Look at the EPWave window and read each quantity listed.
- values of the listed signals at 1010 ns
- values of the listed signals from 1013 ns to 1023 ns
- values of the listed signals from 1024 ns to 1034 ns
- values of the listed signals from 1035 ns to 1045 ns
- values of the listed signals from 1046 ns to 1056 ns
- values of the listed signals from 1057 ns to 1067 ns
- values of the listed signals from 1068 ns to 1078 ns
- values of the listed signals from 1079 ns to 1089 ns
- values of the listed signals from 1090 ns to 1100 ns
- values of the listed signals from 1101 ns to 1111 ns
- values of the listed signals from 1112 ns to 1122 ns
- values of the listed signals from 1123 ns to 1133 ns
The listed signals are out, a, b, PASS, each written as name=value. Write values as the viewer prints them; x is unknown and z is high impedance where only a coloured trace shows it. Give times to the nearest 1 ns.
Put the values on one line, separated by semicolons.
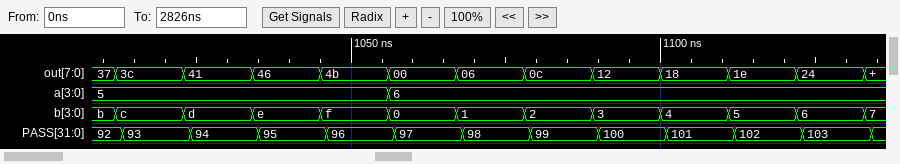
out=37, a=5, b=b, PASS=92; out=3c, a=5, b=c, PASS=93; out=41, a=5, b=d, PASS=94; out=46, a=5, b=e, PASS=95; out=4b, a=5, b=f, PASS=96; out=00, a=6, b=0, PASS=97; out=06, a=6, b=1, PASS=98; out=0c, a=6, b=2, PASS=99; out=12, a=6, b=3, PASS=100; out=18, a=6, b=4, PASS=101; out=1e, a=6, b=5, PASS=102; out=24, a=6, b=6, PASS=103
